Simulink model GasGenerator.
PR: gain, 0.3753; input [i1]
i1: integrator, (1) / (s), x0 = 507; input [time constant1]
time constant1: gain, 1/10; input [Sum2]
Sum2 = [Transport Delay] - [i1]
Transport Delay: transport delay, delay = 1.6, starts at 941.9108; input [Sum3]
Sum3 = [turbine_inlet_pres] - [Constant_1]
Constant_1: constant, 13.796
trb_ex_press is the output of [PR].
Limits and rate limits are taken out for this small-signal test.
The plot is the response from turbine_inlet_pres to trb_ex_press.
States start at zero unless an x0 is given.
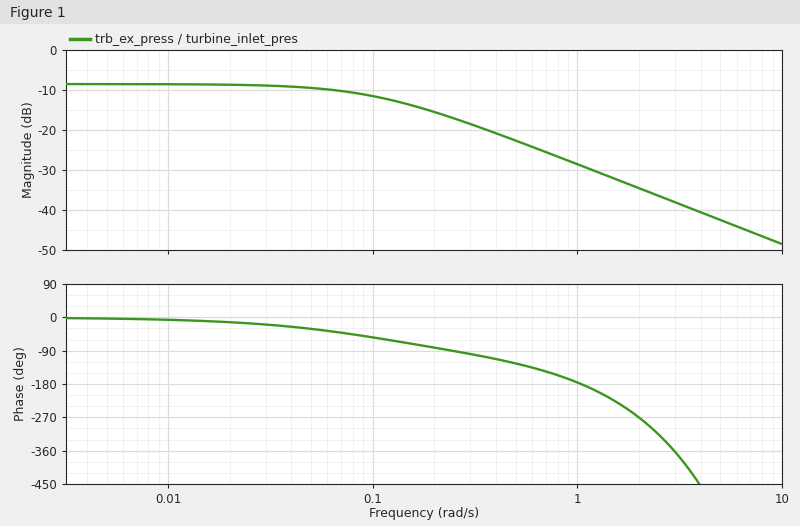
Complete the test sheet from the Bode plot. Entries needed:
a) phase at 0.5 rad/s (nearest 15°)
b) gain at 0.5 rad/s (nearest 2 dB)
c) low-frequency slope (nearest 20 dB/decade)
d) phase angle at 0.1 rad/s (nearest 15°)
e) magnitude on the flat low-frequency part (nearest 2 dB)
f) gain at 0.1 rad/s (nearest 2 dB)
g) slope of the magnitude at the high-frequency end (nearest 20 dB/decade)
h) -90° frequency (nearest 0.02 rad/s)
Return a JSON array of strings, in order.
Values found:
["-120°", "-22 dB", "0 dB/decade", "-60°", "-8 dB", "-12 dB", "-20 dB/decade", "0.24 rad/s"]
